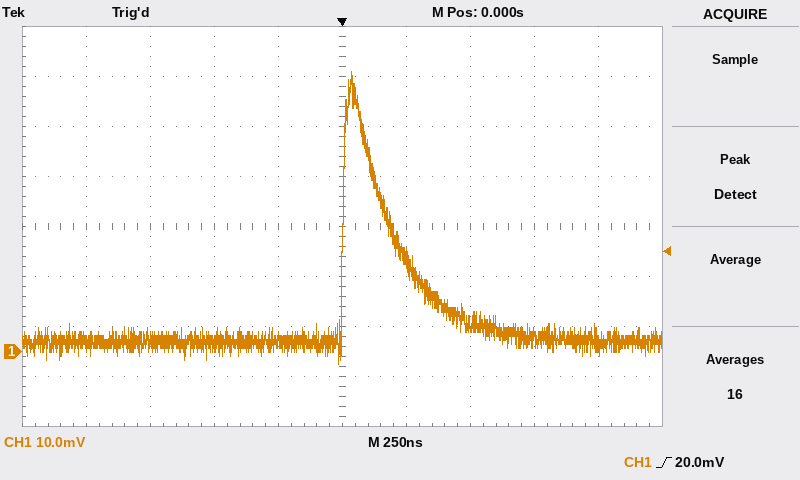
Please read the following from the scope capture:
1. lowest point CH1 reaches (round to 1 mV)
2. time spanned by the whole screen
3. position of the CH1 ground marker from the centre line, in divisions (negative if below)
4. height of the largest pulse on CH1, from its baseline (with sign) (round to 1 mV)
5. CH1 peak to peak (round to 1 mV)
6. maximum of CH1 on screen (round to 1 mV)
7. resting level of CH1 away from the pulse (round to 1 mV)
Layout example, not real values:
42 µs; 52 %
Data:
-2 mV; 2.5 µs; -2.5 div; +54 mV; 58 mV; 56 mV; 2 mV
